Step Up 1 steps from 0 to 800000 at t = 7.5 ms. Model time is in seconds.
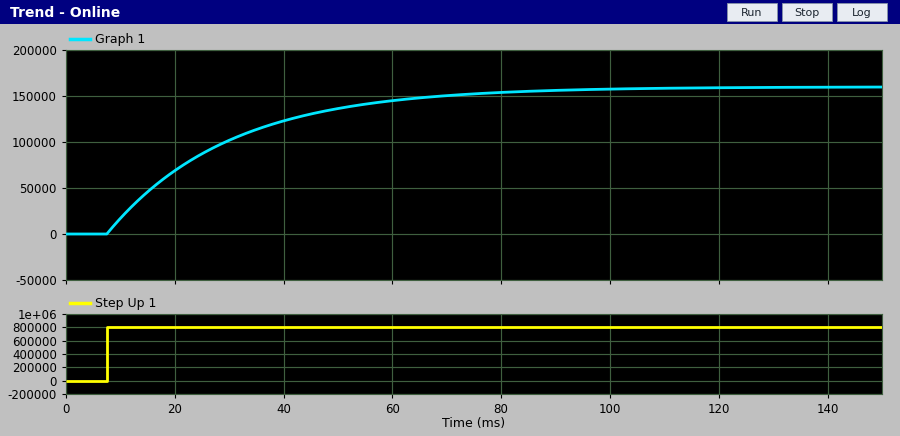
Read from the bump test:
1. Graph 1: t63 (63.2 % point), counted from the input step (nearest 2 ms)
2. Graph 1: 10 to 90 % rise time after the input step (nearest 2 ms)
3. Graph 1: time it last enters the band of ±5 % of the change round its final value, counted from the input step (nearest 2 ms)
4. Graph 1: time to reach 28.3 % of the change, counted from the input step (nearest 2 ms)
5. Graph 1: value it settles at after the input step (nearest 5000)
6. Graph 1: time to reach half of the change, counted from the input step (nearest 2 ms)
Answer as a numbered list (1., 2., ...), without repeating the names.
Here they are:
1. 22 ms
2. 48 ms
3. 66 ms
4. 8 ms
5. 160000
6. 16 ms
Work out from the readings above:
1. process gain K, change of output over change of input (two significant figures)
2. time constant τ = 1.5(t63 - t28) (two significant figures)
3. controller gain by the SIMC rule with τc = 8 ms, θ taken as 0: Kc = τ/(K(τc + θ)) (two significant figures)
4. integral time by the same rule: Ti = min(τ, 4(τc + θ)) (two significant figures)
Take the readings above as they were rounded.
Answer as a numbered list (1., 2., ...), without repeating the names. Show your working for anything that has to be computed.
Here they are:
1. (160000 - 0) / 800000 = 0.20
2. 1.5 × (22 - 8) = 21 ms
3. 21 / (0.2 × (8 + 0)) = 13
4. min(21, 4 × (8 + 0)) = 21 ms
